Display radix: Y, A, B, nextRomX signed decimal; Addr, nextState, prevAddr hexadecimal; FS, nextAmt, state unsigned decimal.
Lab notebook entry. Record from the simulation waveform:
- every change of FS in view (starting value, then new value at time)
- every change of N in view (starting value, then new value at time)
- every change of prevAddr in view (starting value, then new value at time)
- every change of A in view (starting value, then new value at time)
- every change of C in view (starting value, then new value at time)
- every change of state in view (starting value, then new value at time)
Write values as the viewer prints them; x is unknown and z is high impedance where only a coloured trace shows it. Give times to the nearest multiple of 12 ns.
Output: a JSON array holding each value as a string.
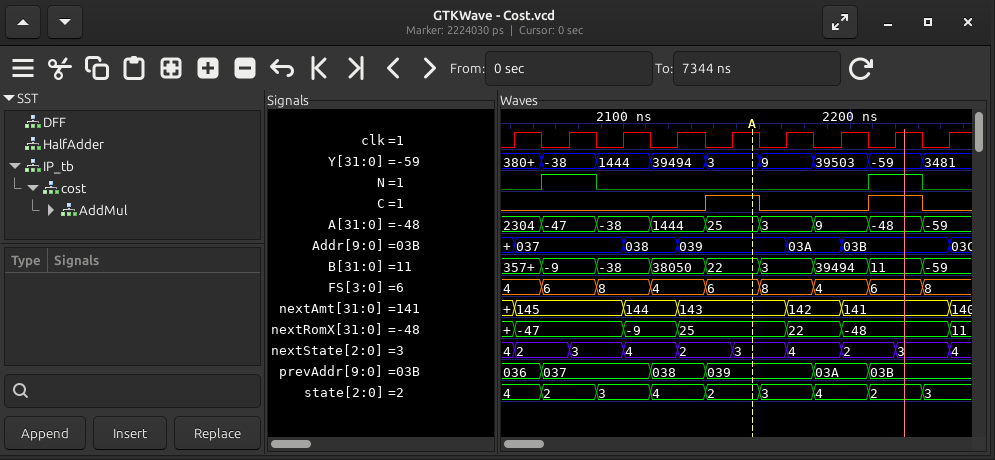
["4, 6 at 2064 ns, 8 at 2088 ns, 4 at 2112 ns, 6 at 2136 ns, 8 at 2160 ns, 4 at 2184 ns, 6 at 2208 ns, 8 at 2232 ns", "0, 1 at 2064 ns, 0 at 2088 ns, 1 at 2208 ns, 0 at 2232 ns", "036, 037 at 2064 ns, 038 at 2112 ns, 039 at 2136 ns, 03A at 2184 ns, 03B at 2208 ns", "2304, -47 at 2064 ns, -38 at 2088 ns, 1444 at 2112 ns, 25 at 2136 ns, 3 at 2160 ns, 9 at 2184 ns, -48 at 2208 ns, -59 at 2232 ns", "0, 1 at 2136 ns, 0 at 2160 ns, 1 at 2208 ns, 0 at 2232 ns", "4, 2 at 2064 ns, 3 at 2088 ns, 4 at 2112 ns, 2 at 2136 ns, 3 at 2160 ns, 4 at 2184 ns, 2 at 2208 ns, 3 at 2232 ns"]
